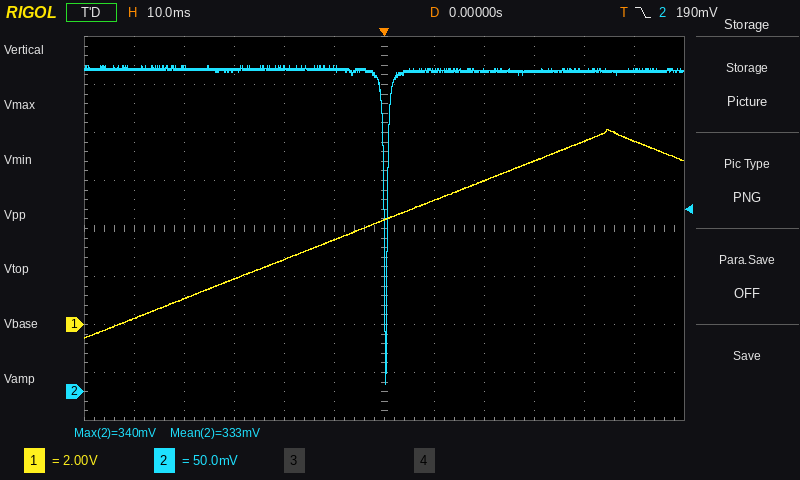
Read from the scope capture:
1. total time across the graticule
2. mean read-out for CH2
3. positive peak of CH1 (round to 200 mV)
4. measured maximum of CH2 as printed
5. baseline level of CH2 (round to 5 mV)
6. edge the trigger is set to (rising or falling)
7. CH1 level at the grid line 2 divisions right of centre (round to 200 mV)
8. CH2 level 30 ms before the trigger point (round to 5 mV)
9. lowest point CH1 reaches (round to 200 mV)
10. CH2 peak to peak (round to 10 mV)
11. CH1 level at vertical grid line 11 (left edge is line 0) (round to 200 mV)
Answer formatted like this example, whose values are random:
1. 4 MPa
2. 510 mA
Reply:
1. 120 ms
2. 333 mV
3. 8.2 V
4. 340 mV
5. 335 mV
6. falling
7. 6.0 V
8. 335 mV
9. -600 mV
10. 330 mV
11. 7.6 V
